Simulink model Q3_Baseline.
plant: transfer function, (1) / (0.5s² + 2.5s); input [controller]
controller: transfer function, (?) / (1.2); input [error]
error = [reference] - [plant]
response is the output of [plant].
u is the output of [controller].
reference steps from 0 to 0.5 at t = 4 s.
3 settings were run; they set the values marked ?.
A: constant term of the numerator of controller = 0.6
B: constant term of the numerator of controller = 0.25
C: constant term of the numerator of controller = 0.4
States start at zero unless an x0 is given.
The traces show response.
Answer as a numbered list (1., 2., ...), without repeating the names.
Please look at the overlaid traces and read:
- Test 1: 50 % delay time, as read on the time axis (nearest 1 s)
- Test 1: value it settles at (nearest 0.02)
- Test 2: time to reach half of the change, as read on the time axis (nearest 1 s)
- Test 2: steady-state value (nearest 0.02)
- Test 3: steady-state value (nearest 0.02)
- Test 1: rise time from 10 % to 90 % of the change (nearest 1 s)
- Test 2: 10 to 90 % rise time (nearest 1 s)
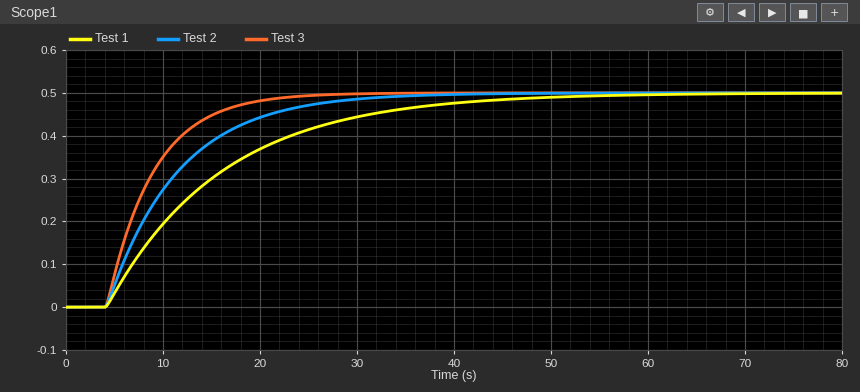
1. 12 s
2. 0.50
3. 9 s
4. 0.50
5. 0.50
6. 26 s
7. 16 s
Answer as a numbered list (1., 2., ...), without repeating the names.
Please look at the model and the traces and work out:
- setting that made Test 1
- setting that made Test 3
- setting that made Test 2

1. B
2. A
3. C
